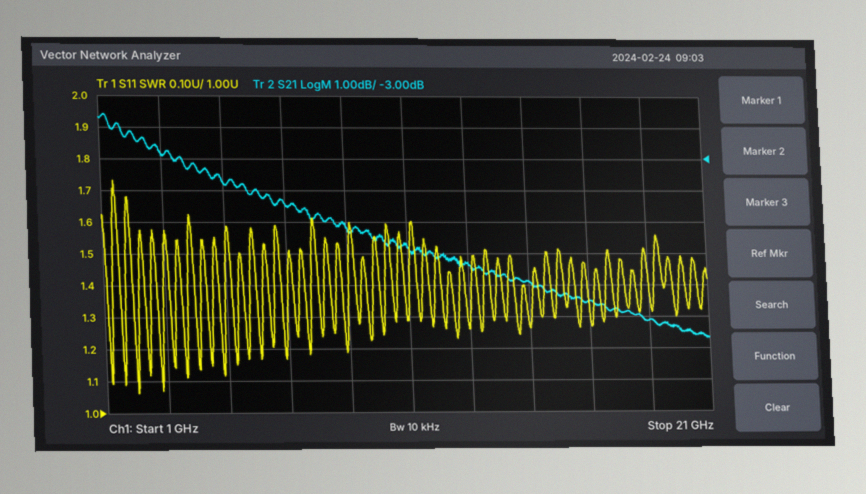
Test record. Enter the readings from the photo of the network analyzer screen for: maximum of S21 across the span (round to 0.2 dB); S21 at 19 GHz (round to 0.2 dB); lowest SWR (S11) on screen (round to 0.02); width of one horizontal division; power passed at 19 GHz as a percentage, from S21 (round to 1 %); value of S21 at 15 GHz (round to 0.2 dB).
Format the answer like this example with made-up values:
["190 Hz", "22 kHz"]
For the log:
["-1.6 dB", "-8.2 dB", "1.06", "2 GHz", "15 %", "-6.8 dB"]
